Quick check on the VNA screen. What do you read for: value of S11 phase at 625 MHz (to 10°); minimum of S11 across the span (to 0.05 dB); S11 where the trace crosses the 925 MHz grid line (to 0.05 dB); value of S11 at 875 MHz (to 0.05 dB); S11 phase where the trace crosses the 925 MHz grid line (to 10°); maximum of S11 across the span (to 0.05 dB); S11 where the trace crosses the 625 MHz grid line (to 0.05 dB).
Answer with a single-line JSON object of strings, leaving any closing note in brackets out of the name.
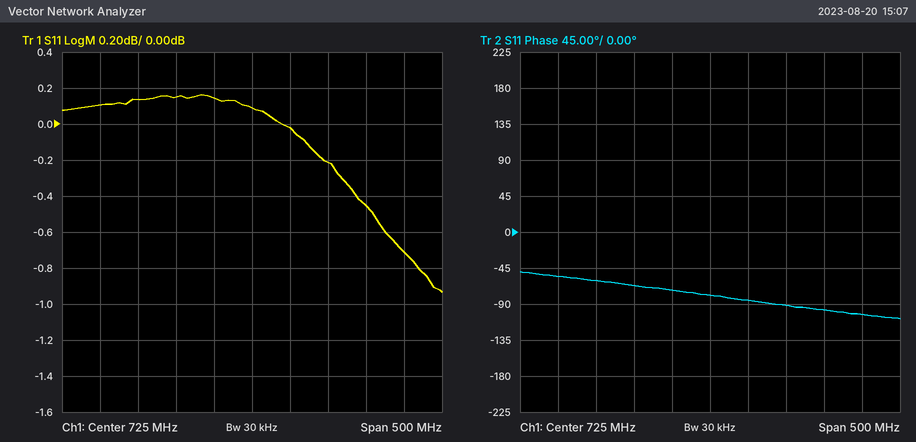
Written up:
{"value of S11 phase at 625 MHz": "-70°", "minimum of S11 across the span": "-0.95 dB", "S11 where the trace crosses the 925 MHz grid line": "-0.70 dB", "value of S11 at 875 MHz": "-0.45 dB", "S11 phase where the trace crosses the 925 MHz grid line": "-100°", "maximum of S11 across the span": "0.15 dB", "S11 where the trace crosses the 625 MHz grid line": "0.15 dB"}
